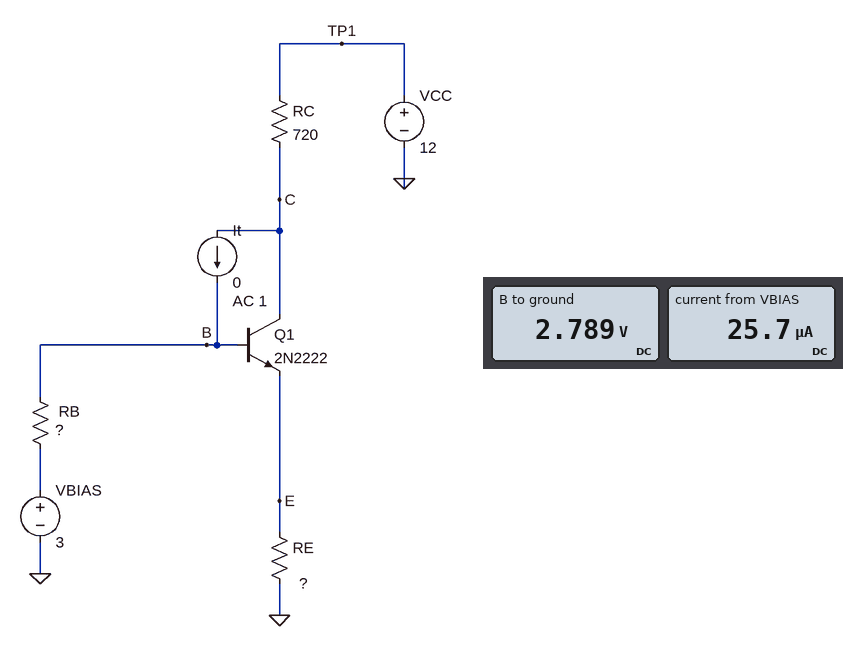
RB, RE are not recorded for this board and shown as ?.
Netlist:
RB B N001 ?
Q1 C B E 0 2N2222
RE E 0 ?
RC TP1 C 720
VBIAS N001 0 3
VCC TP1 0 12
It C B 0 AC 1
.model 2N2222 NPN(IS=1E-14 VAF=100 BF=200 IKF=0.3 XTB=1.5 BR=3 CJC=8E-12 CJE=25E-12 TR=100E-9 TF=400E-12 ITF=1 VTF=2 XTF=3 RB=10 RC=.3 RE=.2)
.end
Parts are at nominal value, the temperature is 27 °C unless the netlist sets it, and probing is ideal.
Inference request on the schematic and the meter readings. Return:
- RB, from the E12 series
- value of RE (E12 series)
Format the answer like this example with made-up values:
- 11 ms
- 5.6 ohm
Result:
- 8.2 kΩ
- 390 Ω
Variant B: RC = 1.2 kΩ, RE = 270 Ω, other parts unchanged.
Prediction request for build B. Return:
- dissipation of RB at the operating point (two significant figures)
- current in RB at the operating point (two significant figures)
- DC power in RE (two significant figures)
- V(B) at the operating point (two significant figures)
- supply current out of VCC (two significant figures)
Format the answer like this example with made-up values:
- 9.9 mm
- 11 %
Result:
- 11 µW
- 37 µA
- 15 mW
- 2.7 V
- 7.3 mA
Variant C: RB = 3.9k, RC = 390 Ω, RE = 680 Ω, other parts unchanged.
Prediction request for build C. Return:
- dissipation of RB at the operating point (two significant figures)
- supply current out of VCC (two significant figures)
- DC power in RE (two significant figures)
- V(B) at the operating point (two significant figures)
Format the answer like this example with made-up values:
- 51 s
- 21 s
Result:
- 930 nW
- 3.3 mA
- 7.5 mW
- 2.9 V
